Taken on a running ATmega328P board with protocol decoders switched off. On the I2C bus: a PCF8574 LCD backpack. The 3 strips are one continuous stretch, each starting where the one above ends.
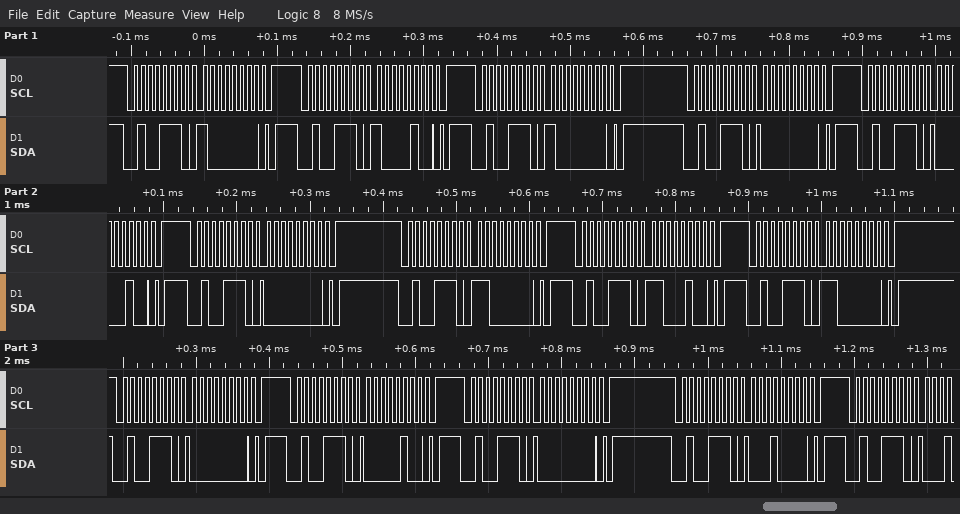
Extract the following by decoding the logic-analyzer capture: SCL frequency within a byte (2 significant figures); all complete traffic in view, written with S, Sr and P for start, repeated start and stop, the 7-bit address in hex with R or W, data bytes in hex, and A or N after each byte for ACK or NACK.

100 kHz
S 27W A 80 A P S 27W A 84 A P S 27W A 80 A P S 27W A 00 A P S 27W A 04 A P S 27W A 00 A P S 27W A C0 A P S 27W A C4 A P S 27W A C0 A P S 27W A 00 A P S 27W A 04 A P S 27W A 00 A P S 27W A 10 A P S 27W A
